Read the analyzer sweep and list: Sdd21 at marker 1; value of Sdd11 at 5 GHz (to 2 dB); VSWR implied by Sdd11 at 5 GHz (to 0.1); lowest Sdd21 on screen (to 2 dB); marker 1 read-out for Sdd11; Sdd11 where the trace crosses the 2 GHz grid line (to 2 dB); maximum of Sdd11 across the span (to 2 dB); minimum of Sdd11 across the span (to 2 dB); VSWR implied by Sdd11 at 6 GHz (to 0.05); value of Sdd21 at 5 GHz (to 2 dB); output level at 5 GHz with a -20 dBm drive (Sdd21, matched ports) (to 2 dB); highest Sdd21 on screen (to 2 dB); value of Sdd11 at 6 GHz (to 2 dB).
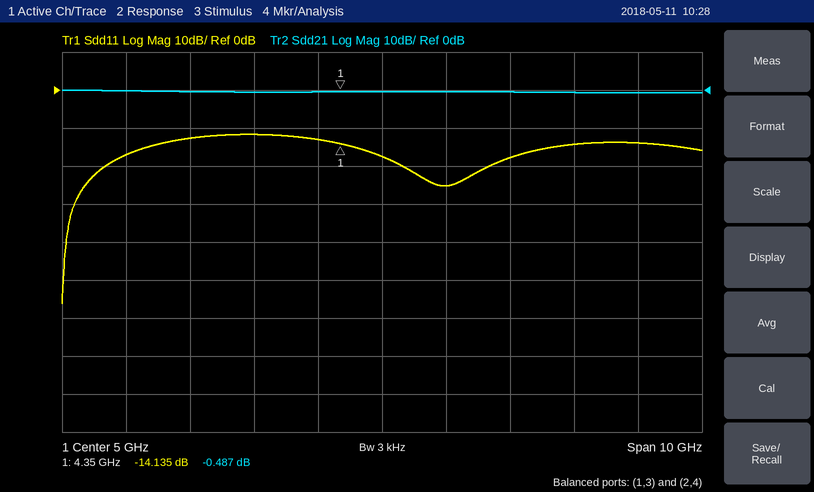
-0.487 dB
-18 dB
1.3
0 dB
-14.135 dB
-12 dB
-12 dB
-56 dB
1.10
0 dB
-20 dBm
0 dB
-26 dB
